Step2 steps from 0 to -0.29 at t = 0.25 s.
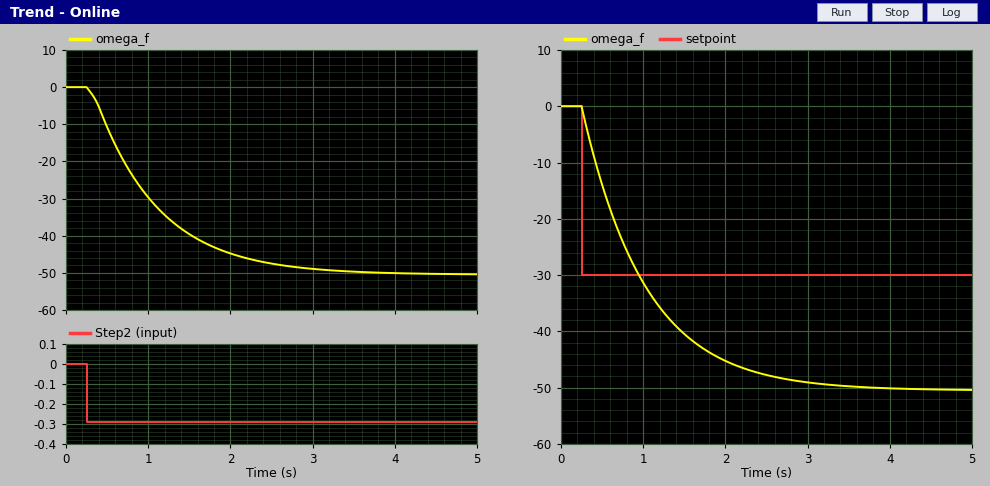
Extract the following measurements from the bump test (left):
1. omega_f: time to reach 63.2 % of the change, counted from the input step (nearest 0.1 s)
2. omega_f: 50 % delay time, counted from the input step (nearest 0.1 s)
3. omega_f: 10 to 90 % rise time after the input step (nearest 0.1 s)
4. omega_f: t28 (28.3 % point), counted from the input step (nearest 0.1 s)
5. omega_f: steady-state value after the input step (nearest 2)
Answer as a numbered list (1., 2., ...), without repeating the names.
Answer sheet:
1. 0.8 s
2. 0.6 s
3. 1.7 s
4. 0.3 s
5. -50
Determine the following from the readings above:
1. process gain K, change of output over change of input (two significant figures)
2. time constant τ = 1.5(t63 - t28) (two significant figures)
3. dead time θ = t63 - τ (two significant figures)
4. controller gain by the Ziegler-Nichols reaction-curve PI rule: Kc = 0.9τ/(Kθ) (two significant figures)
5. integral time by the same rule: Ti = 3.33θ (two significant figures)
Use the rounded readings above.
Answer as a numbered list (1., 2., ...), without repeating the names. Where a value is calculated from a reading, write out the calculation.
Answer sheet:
1. (-50 - 0) / (-0.29) = 170
2. 1.5 × (0.8 - 0.3) = 0.75 s
3. 0.8 - 0.75 = 0.050 s
4. 0.9 × 0.75 / (170 × 0.05) = 0.079
5. 3.33 × 0.05 = 0.17 s
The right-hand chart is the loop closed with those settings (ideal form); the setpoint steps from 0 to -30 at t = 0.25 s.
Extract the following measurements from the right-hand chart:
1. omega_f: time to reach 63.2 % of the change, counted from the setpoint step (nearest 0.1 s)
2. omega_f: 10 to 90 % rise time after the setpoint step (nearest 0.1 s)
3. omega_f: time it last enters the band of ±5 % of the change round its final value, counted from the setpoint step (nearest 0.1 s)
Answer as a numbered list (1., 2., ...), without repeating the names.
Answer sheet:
1. 0.8 s
2. 1.7 s
3. 2.3 s
